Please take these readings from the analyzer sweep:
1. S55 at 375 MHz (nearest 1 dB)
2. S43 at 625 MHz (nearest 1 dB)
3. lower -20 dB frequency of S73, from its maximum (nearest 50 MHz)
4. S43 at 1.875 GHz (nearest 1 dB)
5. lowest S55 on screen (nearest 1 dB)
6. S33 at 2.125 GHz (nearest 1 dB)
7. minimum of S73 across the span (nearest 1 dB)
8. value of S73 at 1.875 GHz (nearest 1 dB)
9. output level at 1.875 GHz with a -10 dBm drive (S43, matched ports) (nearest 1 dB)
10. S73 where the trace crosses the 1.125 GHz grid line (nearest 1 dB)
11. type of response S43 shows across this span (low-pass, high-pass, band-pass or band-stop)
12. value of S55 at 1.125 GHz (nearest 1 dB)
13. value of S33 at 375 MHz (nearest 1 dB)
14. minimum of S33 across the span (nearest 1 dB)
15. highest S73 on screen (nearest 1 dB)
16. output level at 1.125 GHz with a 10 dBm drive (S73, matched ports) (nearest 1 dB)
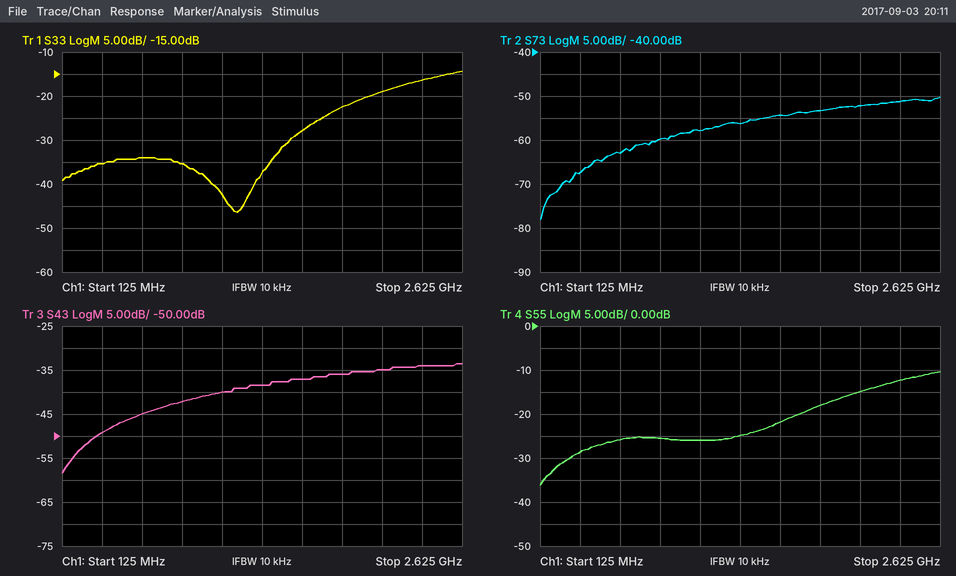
-29 dB
-45 dB
250 MHz
-36 dB
-36 dB
-19 dB
-78 dB
-53 dB
-46 dBm
-58 dB
high-pass
-26 dB
-35 dB
-46 dB
-50 dB
-48 dBm
